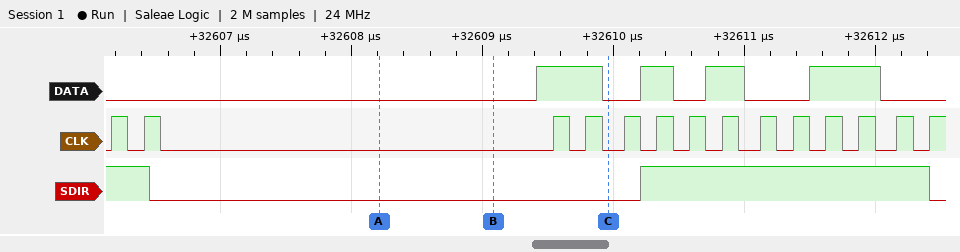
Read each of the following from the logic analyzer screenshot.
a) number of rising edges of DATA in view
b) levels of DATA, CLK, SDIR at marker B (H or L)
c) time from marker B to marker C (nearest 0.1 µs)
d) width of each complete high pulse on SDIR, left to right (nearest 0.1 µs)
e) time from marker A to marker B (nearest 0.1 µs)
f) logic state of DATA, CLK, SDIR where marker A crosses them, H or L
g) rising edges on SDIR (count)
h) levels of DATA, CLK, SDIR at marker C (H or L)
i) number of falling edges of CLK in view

4
DATA=L, CLK=L, SDIR=L
0.9 µs
2.2 µs
0.9 µs
DATA=L, CLK=L, SDIR=L
1
DATA=L, CLK=L, SDIR=L
13
